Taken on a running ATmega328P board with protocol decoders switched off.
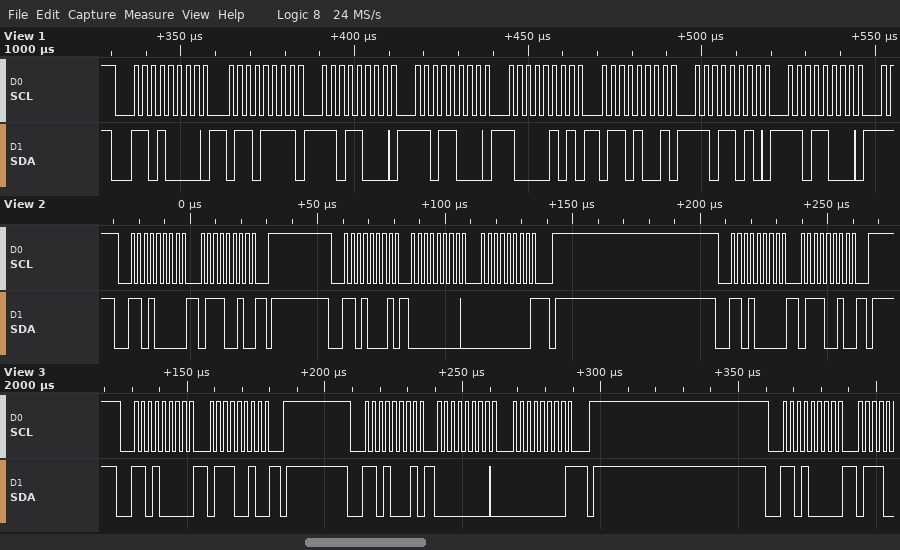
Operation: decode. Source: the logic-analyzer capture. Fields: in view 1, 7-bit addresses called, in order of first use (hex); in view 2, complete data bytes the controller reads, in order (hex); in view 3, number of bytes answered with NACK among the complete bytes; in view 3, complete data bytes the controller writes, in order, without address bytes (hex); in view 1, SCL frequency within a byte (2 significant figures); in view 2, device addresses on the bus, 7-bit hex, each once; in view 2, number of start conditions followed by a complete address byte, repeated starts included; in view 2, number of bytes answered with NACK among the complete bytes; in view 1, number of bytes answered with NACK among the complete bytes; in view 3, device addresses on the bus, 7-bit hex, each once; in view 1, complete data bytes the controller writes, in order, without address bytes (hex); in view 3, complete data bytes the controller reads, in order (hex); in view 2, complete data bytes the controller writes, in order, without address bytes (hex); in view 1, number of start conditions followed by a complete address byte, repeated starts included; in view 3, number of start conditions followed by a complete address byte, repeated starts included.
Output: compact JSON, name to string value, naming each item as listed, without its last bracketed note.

{"in view 1, 7-bit addresses called, in order of first use": "0x68", "in view 2, complete data bytes the controller reads, in order": "00 00", "in view 3, number of bytes answered with NACK among the complete bytes": "1", "in view 3, complete data bytes the controller writes, in order, without address bytes": "72", "in view 1, SCL frequency within a byte": "400 kHz", "in view 2, device addresses on the bus, 7-bit hex, each once": "0x68", "in view 2, number of start conditions followed by a complete address byte, repeated starts included": "3", "in view 2, number of bytes answered with NACK among the complete bytes": "1", "in view 1, number of bytes answered with NACK among the complete bytes": "0", "in view 3, device addresses on the bus, 7-bit hex, each once": "0x68", "in view 1, complete data bytes the controller writes, in order, without address bytes": "6F D8 D8 85 69 DA D8", "in view 3, complete data bytes the controller reads, in order": "00 00", "in view 2, complete data bytes the controller writes, in order, without address bytes": "72 72", "in view 1, number of start conditions followed by a complete address byte, repeated starts included": "1", "in view 3, number of start conditions followed by a complete address byte, repeated starts included": "3"}
